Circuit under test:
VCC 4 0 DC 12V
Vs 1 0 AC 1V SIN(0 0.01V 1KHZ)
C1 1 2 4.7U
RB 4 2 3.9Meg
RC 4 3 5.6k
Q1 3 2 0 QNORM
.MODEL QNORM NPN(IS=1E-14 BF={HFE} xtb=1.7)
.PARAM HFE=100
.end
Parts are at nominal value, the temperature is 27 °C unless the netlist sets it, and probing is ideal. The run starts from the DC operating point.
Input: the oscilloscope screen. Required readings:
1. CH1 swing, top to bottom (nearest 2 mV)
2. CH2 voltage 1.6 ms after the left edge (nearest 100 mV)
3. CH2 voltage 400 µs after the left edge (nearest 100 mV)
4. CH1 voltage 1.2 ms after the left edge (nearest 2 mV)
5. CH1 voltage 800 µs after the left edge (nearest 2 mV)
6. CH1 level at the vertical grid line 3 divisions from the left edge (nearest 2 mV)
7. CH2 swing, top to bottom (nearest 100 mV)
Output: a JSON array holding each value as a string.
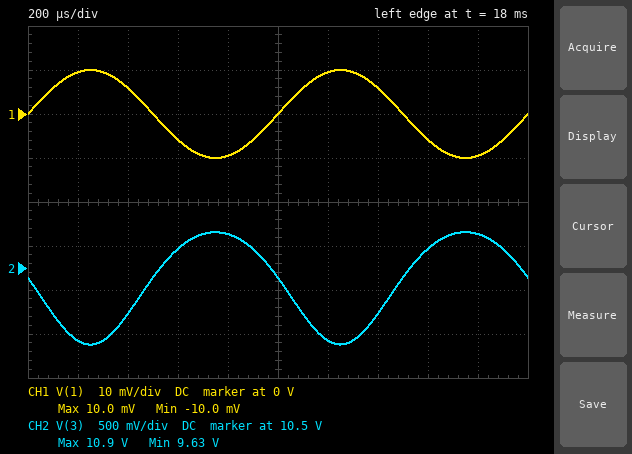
["20 mV", "10.7 V", "10.0 V", "10 mV", "-10 mV", "-6 mV", "1.3 V"]
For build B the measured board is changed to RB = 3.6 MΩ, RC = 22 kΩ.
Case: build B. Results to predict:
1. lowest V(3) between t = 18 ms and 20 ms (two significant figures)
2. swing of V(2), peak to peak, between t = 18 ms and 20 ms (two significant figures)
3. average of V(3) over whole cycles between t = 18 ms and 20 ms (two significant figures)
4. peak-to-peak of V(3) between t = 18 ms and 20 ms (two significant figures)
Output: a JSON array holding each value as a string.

["1.9 V", "20 mV", "4.9 V", "5.4 V"]
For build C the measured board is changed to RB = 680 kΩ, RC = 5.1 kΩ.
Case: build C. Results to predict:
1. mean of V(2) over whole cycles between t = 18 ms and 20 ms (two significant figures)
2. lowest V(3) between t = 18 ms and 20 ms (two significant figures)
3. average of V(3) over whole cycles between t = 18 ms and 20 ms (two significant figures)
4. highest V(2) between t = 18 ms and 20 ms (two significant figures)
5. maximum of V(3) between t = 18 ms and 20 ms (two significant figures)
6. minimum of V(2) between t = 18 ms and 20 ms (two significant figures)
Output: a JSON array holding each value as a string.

["670 mV", "160 mV", "3.6 V", "680 mV", "6.5 V", "660 mV"]
